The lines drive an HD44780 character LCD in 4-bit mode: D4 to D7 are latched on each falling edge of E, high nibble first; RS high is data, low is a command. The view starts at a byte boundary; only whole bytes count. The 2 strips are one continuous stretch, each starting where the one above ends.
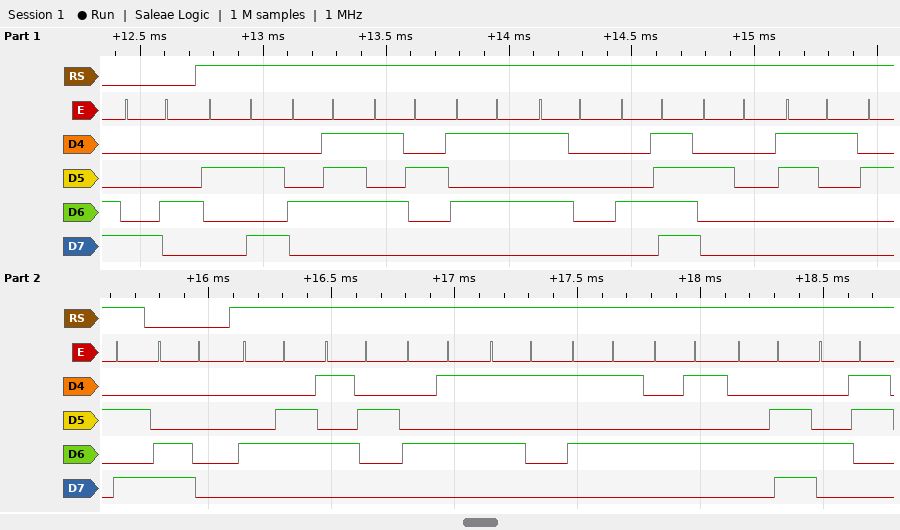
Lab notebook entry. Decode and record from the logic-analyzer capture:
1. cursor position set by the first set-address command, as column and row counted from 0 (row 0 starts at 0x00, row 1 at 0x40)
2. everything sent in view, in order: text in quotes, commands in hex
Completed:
column 4, row 0
0x84 "*GRUPO 1*" 0xC0 "FREQUENC"
